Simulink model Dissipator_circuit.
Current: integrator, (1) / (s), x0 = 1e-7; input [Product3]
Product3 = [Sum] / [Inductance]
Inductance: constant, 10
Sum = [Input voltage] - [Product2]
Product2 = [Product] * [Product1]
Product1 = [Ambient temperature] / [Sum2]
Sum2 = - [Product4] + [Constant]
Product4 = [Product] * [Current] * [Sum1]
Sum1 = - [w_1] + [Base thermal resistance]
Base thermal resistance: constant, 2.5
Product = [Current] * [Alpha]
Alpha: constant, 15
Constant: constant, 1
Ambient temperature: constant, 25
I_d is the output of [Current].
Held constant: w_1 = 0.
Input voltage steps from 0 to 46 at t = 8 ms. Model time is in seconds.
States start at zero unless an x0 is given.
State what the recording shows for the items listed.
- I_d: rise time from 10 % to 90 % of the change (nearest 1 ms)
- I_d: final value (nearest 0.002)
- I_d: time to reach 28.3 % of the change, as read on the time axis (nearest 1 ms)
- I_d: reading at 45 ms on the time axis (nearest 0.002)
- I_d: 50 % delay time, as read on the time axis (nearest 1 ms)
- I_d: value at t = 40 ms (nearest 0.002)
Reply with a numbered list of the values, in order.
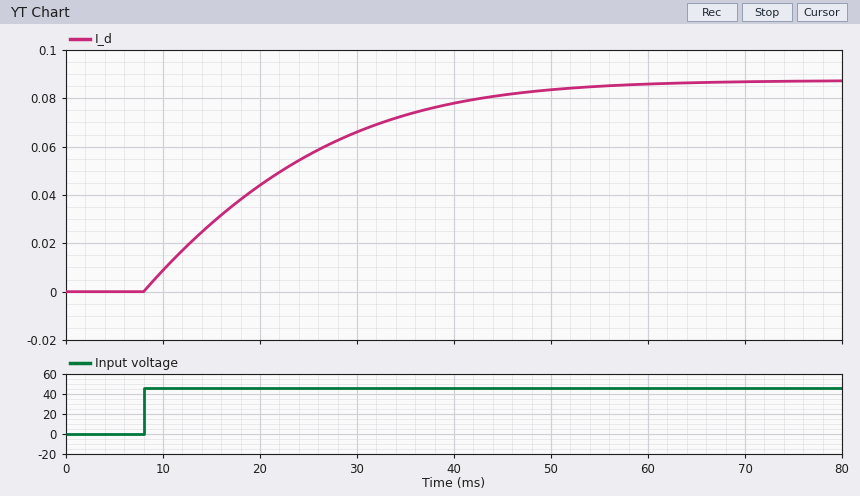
1. 31 ms
2. 0.088
3. 14 ms
4. 0.082
5. 20 ms
6. 0.078
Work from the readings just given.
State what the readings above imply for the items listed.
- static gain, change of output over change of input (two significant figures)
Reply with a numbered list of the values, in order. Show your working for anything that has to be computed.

1. (0.088 - 0) / (46 - 0) = 0.0019
